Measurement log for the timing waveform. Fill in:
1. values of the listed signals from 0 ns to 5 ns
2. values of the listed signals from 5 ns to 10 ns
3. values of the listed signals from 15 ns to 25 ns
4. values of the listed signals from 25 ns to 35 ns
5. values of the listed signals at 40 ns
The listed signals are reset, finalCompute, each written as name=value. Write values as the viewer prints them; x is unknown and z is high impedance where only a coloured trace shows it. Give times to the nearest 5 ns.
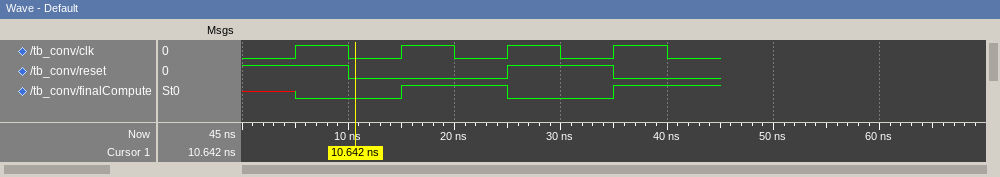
reset=1, finalCompute=x
reset=1, finalCompute=0
reset=0, finalCompute=1
reset=1, finalCompute=0
reset=0, finalCompute=1
